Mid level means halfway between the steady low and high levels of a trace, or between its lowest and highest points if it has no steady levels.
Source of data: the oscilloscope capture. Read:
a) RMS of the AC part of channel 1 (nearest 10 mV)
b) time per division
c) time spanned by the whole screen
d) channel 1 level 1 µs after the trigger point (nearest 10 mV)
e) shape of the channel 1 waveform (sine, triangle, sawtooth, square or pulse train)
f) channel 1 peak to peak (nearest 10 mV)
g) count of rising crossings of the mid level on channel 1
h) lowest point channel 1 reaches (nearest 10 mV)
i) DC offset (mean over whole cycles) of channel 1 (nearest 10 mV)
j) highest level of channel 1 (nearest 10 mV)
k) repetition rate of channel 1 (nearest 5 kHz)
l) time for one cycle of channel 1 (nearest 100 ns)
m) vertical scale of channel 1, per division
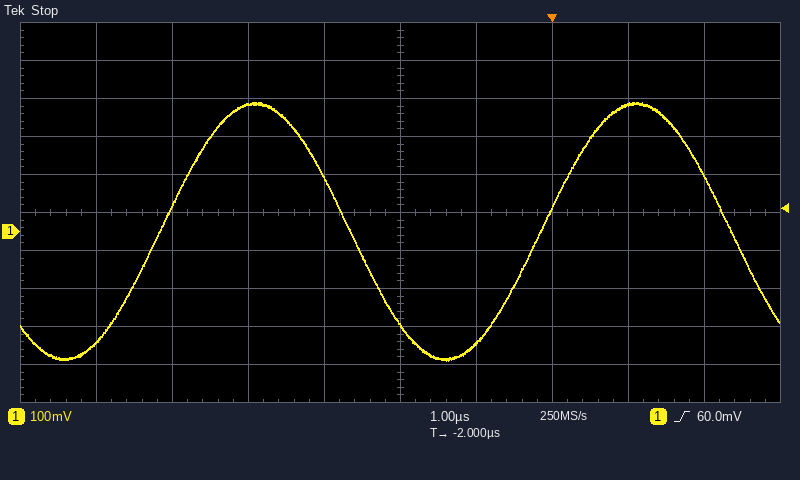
240 mV
1 µs
10 µs
330 mV
sine
680 mV
2
-340 mV
0 mV
340 mV
200 kHz
5.0 µs
100 mV
